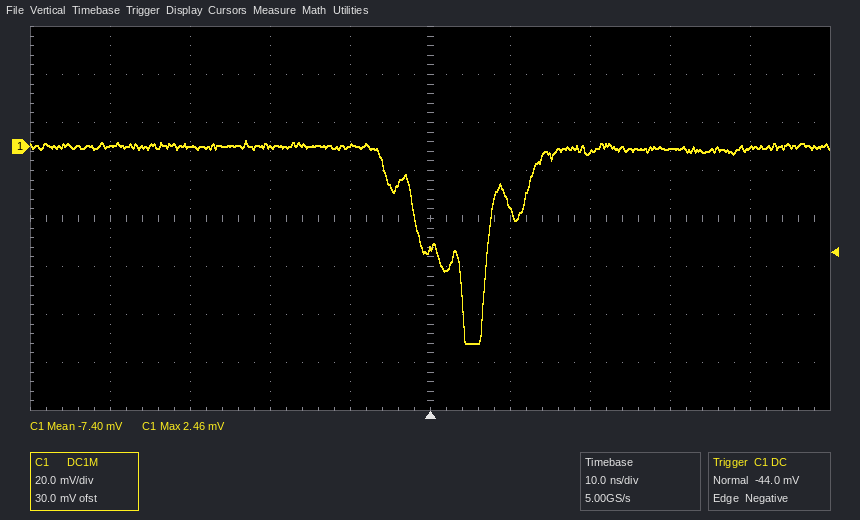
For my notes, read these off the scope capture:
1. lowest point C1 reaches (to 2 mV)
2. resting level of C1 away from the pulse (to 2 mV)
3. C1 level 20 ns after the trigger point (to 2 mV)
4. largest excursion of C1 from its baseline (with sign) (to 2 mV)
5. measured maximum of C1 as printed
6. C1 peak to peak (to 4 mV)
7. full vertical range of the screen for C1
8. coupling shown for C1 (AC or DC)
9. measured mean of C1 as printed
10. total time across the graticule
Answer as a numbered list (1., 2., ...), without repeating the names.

1. -82 mV
2. 0 mV
3. -2 mV
4. -82 mV
5. 2.46 mV
6. 84 mV
7. 160 mV
8. DC
9. -7.40 mV
10. 100 ns
